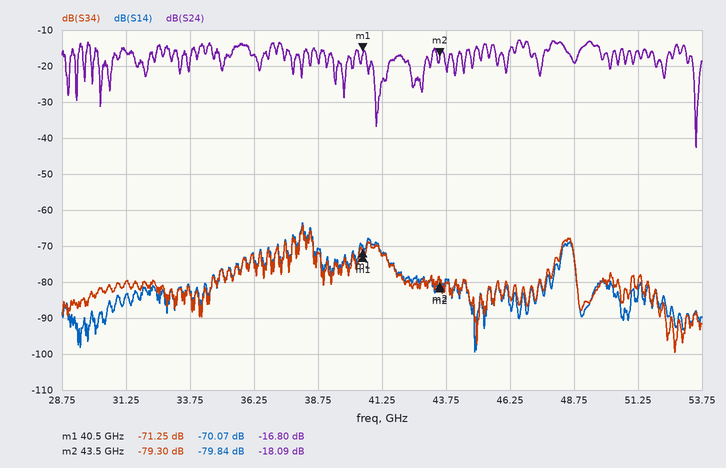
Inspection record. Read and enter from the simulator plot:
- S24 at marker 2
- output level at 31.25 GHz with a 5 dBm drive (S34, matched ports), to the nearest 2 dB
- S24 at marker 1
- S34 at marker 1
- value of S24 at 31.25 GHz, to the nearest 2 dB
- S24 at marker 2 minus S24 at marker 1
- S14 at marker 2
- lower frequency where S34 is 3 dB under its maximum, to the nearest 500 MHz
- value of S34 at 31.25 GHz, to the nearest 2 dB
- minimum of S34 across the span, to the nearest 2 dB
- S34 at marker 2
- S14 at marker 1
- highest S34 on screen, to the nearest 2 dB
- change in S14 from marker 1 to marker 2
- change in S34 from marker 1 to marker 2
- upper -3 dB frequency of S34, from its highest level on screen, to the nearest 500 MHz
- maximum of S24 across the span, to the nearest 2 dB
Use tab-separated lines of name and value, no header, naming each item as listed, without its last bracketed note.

S24 at marker 2	-18.09 dB
output level at 31.25 GHz with a 5 dBm drive (S34, matched ports), to the nearest 2 dB	-74 dBm
S24 at marker 1	-16.80 dB
S34 at marker 1	-71.25 dB
value of S24 at 31.25 GHz, to the nearest 2 dB	-16 dB
S24 at marker 2 minus S24 at marker 1	-1.29 dB
S14 at marker 2	-79.84 dB
lower frequency where S34 is 3 dB under its maximum, to the nearest 500 MHz	38.0 GHz
value of S34 at 31.25 GHz, to the nearest 2 dB	-80 dB
minimum of S34 across the span, to the nearest 2 dB	-100 dB
S34 at marker 2	-79.30 dB
S14 at marker 1	-70.07 dB
highest S34 on screen, to the nearest 2 dB	-64 dB
change in S14 from marker 1 to marker 2	-9.77 dB
change in S34 from marker 1 to marker 2	-8.05 dB
upper -3 dB frequency of S34, from its highest level on screen, to the nearest 500 MHz	38.0 GHz
maximum of S24 across the span, to the nearest 2 dB	-12 dB
